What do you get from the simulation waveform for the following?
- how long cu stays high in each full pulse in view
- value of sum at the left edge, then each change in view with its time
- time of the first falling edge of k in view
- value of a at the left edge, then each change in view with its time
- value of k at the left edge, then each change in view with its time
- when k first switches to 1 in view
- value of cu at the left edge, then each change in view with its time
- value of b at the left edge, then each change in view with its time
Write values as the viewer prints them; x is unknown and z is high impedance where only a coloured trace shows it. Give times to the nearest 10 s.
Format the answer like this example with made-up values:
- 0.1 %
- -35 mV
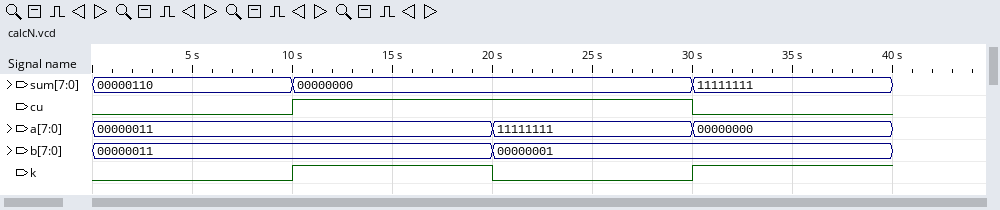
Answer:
- 20 s
- 00000110, 00000000 at 10 s, 11111111 at 30 s
- 20 s
- 00000011, 11111111 at 20 s, 00000000 at 30 s
- 0, 1 at 10 s, 0 at 20 s, 1 at 30 s
- 10 s
- 0, 1 at 10 s, 0 at 30 s
- 00000011, 00000001 at 20 s
